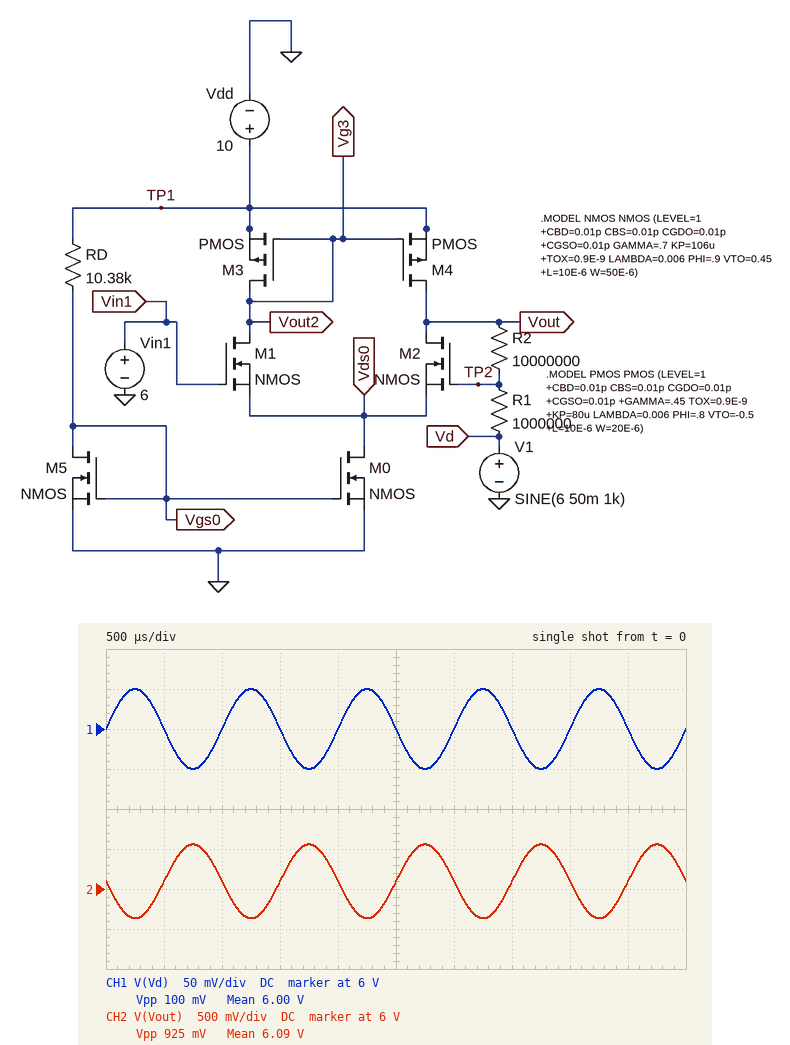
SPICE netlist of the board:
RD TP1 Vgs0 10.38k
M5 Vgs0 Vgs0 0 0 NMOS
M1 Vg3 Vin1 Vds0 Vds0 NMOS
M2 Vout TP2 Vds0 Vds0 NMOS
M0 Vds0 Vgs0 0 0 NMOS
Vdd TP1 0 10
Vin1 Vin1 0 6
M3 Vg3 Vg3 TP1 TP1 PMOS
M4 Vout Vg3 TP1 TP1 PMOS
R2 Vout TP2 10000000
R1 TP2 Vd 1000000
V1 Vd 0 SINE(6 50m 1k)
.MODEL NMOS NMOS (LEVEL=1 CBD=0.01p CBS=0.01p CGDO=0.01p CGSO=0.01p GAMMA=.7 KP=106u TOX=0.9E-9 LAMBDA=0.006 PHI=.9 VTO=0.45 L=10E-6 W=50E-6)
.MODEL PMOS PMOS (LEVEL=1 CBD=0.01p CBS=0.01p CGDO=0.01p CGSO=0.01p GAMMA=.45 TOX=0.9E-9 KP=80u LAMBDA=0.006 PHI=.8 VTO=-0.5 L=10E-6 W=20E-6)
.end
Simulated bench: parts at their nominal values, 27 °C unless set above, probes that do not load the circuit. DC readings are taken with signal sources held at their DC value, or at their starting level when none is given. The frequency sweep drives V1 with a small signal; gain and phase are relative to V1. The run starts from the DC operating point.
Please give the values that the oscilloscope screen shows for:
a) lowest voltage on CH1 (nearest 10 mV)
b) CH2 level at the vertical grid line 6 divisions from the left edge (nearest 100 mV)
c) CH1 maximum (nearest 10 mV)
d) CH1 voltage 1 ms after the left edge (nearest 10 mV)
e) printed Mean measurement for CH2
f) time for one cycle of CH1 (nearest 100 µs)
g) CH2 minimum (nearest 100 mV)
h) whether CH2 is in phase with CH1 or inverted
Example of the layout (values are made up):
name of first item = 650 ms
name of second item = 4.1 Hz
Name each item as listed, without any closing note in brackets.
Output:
lowest voltage on CH1 = 5.95 V
CH2 level at the vertical grid line 6 divisions from the left edge = 6.1 V
CH1 maximum = 6.05 V
CH1 voltage 1 ms after the left edge = 6.00 V
printed Mean measurement for CH2 = 6.09 V
time for one cycle of CH1 = 1.0 ms
CH2 minimum = 5.6 V
whether CH2 is in phase with CH1 or inverted = inverted
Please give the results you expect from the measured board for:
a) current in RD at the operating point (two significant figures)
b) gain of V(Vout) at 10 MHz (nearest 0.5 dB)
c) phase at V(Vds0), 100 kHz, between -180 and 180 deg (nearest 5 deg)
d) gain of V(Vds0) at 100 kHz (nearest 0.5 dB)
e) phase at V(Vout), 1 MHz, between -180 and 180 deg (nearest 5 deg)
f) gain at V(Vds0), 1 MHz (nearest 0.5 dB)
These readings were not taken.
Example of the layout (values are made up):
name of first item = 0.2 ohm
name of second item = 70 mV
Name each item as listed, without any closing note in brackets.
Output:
current in RD at the operating point = 760 µA
gain of V(Vout) at 10 MHz = -12.5 dB
phase at V(Vds0), 100 kHz, between -180 and 180 deg = -20 deg
gain of V(Vds0) at 100 kHz = -36.0 dB
phase at V(Vout), 1 MHz, between -180 and 180 deg = 105 deg
gain at V(Vds0), 1 MHz = -47.5 dB
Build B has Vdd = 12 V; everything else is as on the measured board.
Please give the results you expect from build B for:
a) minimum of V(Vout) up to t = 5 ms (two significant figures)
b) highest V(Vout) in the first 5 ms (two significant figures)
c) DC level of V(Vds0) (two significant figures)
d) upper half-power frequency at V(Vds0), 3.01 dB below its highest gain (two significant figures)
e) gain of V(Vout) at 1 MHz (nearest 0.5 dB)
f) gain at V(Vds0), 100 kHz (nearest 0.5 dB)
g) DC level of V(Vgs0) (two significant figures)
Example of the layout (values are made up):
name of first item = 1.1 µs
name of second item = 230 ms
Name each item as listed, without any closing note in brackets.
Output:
minimum of V(Vout) up to t = 5 ms = 5.8 V
highest V(Vout) in the first 5 ms = 6.7 V
DC level of V(Vds0) = 4.2 V
upper half-power frequency at V(Vds0), 3.01 dB below its highest gain = 230 kHz
gain of V(Vout) at 1 MHz = 6.0 dB
gain at V(Vds0), 100 kHz = -35.5 dB
DC level of V(Vgs0) = 2.3 V
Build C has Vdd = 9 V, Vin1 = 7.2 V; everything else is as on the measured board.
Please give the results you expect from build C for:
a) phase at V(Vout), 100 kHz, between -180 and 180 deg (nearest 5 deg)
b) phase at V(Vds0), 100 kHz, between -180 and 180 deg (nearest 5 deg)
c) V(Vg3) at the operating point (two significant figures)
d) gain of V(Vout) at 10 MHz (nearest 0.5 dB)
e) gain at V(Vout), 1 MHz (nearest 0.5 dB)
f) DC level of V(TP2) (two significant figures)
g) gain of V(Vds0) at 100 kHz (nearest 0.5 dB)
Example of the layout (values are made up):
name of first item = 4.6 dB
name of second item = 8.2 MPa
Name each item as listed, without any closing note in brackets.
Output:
phase at V(Vout), 100 kHz, between -180 and 180 deg = 105 deg
phase at V(Vds0), 100 kHz, between -180 and 180 deg = -75 deg
V(Vg3) at the operating point = 5.9 V
gain of V(Vout) at 10 MHz = -60.0 dB
gain at V(Vout), 1 MHz = -37.0 dB
DC level of V(TP2) = 6.2 V
gain of V(Vds0) at 100 kHz = -19.5 dB
